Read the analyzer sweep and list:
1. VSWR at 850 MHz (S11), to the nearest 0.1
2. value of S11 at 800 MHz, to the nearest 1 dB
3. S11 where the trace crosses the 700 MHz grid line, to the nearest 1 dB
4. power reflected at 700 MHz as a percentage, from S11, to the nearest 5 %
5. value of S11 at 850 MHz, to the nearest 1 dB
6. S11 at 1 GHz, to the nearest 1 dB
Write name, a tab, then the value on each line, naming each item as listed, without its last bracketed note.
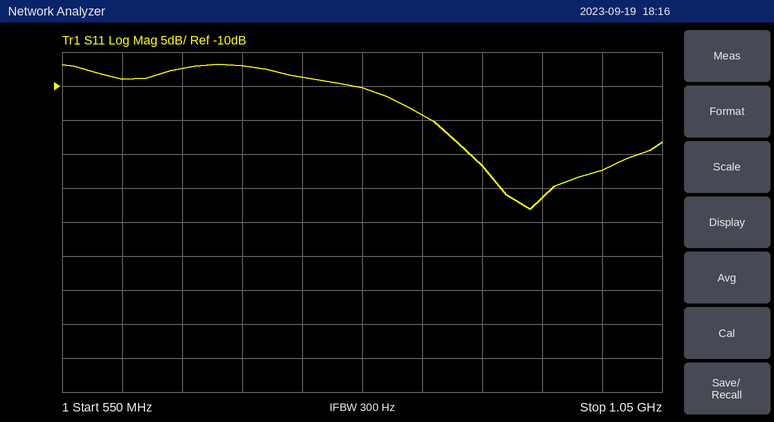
VSWR at 850 MHz (S11), to the nearest 0.1	1.5
value of S11 at 800 MHz, to the nearest 1 dB	-10 dB
S11 where the trace crosses the 700 MHz grid line, to the nearest 1 dB	-7 dB
power reflected at 700 MHz as a percentage, from S11, to the nearest 5 %	20 %
value of S11 at 850 MHz, to the nearest 1 dB	-14 dB
S11 at 1 GHz, to the nearest 1 dB	-22 dB
